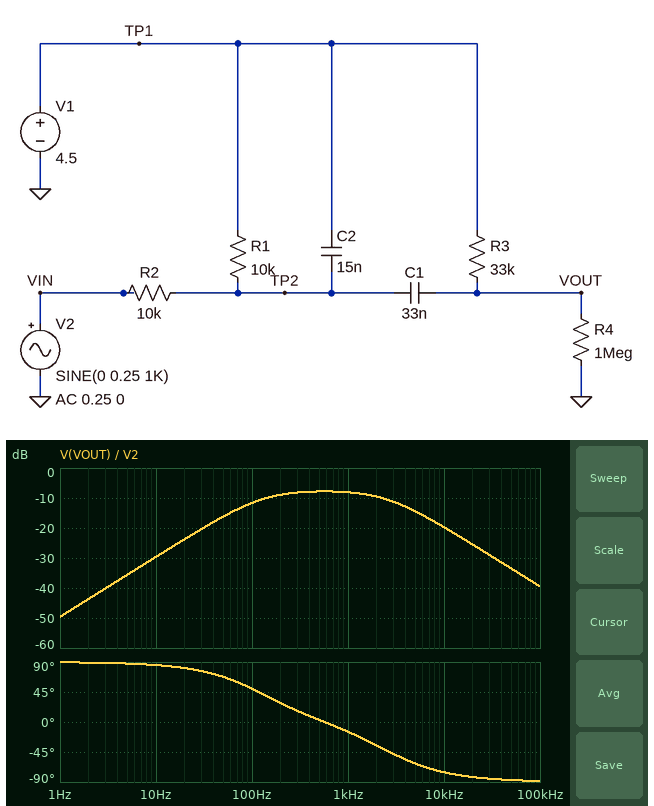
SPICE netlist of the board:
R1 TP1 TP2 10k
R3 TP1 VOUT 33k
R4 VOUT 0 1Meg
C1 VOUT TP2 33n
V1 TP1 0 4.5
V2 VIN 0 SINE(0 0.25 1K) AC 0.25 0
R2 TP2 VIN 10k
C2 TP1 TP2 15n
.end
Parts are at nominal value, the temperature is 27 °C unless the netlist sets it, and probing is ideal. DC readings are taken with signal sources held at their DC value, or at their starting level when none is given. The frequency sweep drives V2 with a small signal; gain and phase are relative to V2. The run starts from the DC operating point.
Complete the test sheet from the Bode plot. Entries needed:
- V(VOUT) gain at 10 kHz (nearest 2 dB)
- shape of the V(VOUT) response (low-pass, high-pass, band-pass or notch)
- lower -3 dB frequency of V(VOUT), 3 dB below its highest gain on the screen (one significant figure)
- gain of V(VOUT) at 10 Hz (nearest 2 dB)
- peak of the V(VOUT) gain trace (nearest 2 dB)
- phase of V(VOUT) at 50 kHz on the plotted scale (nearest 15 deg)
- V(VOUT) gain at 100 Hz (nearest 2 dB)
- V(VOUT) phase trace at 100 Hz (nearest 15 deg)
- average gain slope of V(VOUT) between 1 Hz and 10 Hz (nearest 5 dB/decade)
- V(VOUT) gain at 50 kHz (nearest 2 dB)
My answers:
-20 dB
band-pass
100 Hz
-30 dB
-8 dB
-90 deg
-12 dB
45 deg
20 dB/decade
-34 dB
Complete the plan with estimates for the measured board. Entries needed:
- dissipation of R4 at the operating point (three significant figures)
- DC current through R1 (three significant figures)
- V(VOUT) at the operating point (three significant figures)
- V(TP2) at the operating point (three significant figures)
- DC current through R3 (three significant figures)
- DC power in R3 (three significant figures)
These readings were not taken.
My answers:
19.0 µW
225 µA
4.36 V
2.25 V
4.36 µA
626 nW
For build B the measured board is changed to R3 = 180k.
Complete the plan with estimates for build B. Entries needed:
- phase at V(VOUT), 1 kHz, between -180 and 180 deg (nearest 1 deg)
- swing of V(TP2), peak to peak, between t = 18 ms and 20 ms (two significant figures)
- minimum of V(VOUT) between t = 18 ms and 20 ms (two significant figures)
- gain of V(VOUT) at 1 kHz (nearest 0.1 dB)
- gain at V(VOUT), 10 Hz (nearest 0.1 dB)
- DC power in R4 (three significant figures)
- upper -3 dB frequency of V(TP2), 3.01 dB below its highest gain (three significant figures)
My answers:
-23 deg
220 mV
3.7 V
-7.1 dB
-16.5 dB
14.5 µW
2.05 kHz
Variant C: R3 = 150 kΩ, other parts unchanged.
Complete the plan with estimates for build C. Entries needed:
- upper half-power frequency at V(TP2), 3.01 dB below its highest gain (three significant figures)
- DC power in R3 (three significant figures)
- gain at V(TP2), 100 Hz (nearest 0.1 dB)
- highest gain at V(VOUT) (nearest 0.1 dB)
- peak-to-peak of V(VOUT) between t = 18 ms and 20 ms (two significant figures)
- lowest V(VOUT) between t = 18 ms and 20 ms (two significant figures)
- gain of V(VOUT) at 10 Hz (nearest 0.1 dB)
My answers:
2.04 kHz
2.30 µW
-6.3 dB
-6.5 dB
220 mV
3.8 V
-17.7 dB
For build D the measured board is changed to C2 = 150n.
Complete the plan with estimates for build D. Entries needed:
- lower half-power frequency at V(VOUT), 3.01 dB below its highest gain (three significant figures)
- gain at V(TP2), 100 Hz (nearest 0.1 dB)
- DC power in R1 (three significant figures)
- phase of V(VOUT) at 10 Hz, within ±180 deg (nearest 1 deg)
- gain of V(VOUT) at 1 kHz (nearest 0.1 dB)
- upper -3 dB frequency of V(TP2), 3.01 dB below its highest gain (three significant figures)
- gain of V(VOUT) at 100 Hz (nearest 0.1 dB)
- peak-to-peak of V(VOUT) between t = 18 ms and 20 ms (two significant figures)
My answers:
68.9 Hz
-7.5 dB
506 µW
83 deg
-19.9 dB
175 Hz
-12.6 dB
51 mV
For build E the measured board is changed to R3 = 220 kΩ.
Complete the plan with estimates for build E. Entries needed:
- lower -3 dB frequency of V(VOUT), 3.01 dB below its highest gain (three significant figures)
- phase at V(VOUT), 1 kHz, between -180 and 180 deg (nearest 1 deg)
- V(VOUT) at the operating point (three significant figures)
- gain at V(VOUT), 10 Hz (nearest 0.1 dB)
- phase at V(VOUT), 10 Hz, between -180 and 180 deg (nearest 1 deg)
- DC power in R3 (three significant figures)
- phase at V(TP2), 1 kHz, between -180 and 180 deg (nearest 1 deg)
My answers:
25.4 Hz
-23 deg
3.69 V
-15.2 dB
69 deg
2.99 µW
-25 deg
